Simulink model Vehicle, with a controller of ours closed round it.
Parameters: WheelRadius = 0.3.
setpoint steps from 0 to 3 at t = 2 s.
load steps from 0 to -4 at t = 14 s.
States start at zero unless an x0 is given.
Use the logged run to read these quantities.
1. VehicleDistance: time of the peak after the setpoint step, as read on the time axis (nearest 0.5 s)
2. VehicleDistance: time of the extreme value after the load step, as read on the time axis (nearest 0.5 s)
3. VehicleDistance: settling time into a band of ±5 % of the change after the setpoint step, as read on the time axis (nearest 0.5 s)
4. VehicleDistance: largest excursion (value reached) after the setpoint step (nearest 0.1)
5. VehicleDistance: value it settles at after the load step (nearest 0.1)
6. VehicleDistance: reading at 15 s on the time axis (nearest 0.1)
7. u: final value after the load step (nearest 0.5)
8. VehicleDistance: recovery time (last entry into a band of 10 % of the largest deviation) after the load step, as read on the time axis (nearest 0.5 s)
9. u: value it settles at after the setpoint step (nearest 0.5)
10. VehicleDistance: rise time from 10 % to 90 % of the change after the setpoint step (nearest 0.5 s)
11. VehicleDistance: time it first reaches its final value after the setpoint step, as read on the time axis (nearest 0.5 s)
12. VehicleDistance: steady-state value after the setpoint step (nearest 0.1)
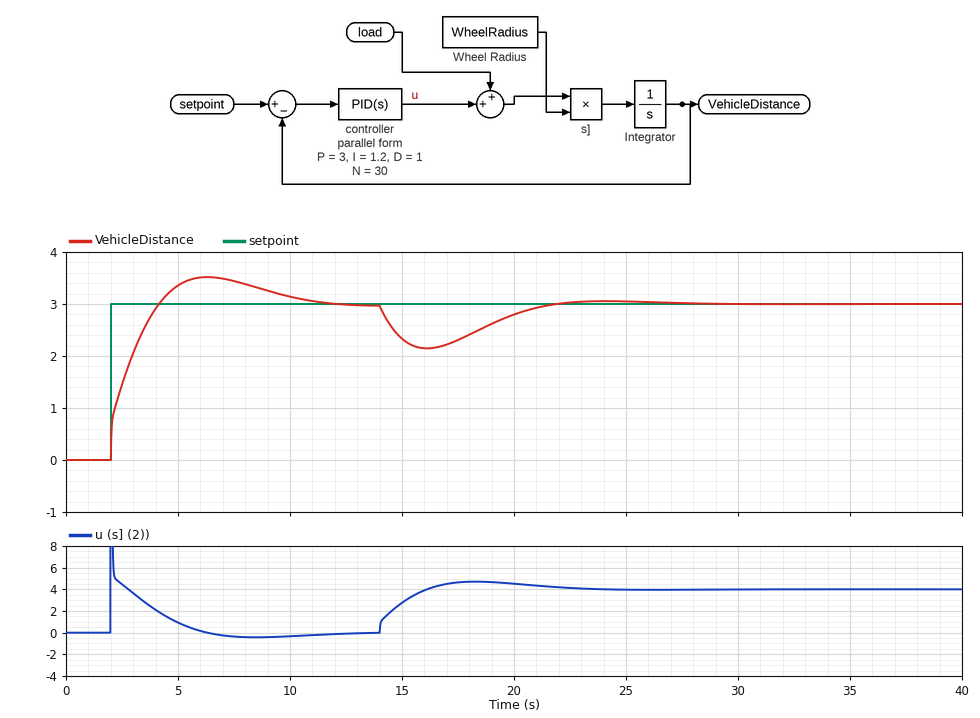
6.5 s
16.0 s
10.0 s
3.5
3.0
2.3
4.0
21.0 s
0.0
1.5 s
4.0 s
3.0
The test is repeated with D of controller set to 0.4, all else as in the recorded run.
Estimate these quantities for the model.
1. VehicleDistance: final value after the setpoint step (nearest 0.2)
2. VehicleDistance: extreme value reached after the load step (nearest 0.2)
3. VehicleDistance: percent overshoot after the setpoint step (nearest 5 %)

3.0
2.2
20 %
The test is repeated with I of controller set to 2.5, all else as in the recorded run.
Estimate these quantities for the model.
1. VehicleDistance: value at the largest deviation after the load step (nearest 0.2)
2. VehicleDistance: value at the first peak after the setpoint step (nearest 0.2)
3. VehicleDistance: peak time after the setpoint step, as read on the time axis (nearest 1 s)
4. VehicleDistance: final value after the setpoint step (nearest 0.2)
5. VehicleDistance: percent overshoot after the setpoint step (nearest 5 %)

2.4
3.8
5 s
3.0
25 %
